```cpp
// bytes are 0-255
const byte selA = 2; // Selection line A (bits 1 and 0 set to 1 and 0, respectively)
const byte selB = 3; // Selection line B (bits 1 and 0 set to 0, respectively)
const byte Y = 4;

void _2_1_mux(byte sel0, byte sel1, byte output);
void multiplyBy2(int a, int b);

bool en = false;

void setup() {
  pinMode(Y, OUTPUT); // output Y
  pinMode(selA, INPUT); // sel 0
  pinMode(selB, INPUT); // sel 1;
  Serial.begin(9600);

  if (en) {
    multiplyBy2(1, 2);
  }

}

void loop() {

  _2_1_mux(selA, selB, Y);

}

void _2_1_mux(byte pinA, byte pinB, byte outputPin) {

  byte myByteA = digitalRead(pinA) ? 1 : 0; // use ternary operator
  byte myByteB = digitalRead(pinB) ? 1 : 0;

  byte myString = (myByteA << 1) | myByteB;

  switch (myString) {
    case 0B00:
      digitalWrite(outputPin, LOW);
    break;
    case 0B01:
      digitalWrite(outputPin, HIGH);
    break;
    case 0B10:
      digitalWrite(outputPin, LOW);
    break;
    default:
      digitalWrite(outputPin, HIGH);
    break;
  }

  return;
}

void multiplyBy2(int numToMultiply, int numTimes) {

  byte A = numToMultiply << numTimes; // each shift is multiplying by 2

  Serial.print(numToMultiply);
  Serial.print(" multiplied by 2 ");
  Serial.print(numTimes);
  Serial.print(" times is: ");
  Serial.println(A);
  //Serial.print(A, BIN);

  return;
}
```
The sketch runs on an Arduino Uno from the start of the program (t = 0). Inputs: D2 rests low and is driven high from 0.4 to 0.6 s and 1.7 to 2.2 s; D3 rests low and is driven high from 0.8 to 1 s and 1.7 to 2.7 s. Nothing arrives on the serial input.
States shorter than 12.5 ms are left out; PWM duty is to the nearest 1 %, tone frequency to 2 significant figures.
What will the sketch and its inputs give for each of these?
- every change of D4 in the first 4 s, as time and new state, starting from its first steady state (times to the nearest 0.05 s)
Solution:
0 s low; 0.8 s high; 1 s low; 1.7 s high; 2.7 s low
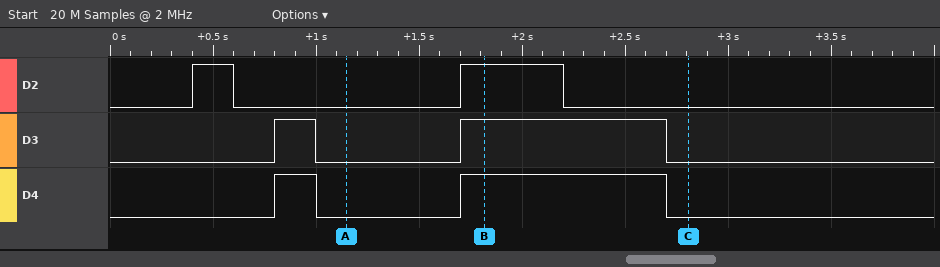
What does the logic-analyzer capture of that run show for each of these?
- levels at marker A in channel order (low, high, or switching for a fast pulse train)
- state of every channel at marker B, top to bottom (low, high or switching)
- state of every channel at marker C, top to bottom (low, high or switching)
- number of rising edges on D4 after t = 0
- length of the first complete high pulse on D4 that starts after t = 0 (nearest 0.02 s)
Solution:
D2 low, D3 low, D4 low
D2 high, D3 high, D4 high
D2 low, D3 low, D4 low
2
0.20 s
